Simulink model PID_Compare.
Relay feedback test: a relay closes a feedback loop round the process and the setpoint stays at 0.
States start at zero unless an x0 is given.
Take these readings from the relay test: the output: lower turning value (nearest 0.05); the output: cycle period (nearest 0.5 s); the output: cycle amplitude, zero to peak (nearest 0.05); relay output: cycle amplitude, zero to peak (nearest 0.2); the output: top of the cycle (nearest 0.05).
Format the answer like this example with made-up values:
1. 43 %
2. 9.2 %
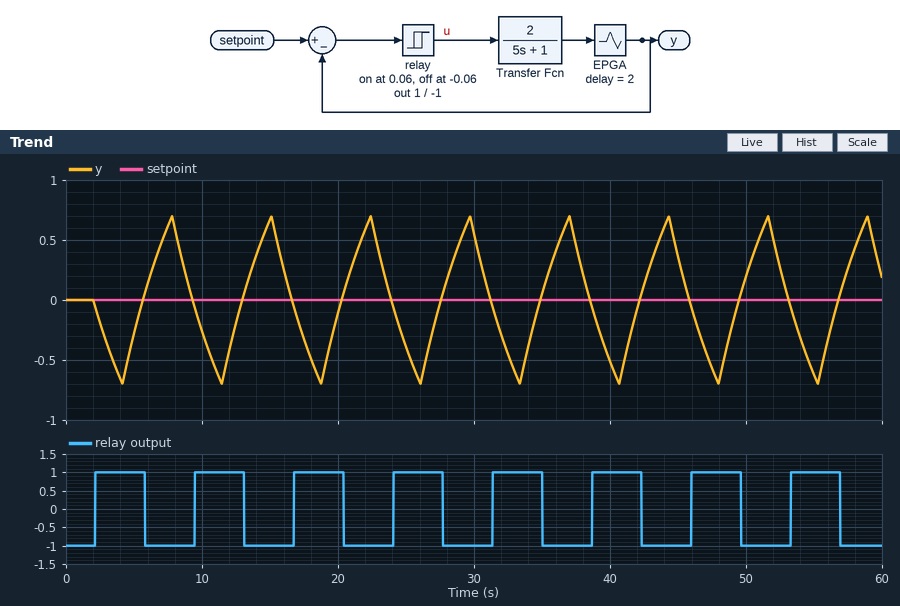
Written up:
1. -0.70
2. 7.5 s
3. 0.70
4. 1.0
5. 0.70
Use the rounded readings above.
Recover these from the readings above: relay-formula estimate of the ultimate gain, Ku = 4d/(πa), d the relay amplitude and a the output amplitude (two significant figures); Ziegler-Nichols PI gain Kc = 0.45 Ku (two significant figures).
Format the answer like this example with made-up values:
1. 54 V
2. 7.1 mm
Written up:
1. 1.8
2. 0.81
